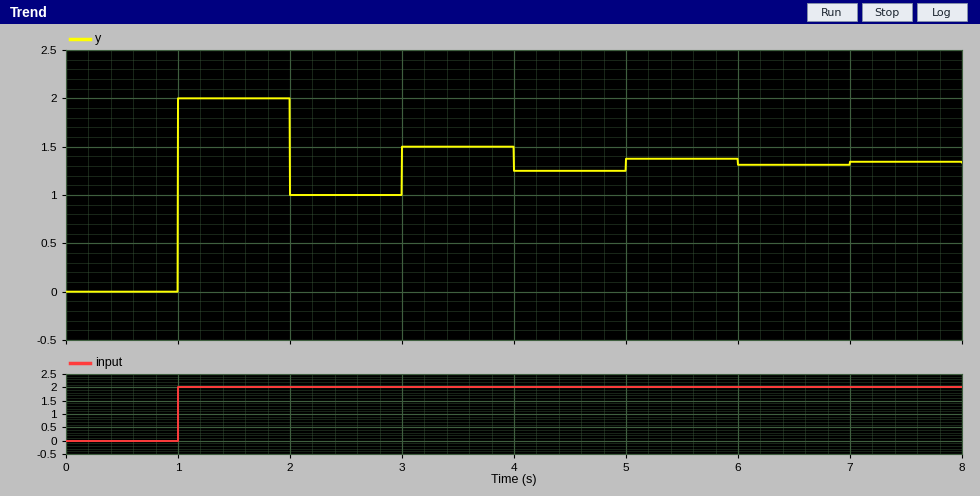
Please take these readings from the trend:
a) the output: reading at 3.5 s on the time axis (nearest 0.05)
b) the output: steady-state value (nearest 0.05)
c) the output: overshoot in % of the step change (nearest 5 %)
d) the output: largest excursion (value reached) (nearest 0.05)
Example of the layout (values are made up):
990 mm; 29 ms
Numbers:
1.50; 1.35; 50 %; 2.00
